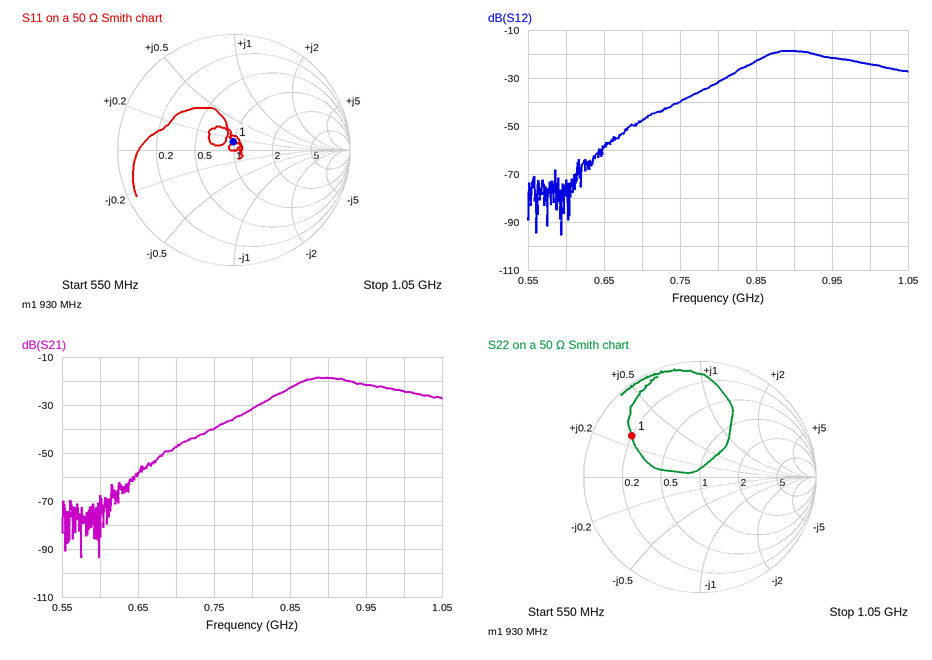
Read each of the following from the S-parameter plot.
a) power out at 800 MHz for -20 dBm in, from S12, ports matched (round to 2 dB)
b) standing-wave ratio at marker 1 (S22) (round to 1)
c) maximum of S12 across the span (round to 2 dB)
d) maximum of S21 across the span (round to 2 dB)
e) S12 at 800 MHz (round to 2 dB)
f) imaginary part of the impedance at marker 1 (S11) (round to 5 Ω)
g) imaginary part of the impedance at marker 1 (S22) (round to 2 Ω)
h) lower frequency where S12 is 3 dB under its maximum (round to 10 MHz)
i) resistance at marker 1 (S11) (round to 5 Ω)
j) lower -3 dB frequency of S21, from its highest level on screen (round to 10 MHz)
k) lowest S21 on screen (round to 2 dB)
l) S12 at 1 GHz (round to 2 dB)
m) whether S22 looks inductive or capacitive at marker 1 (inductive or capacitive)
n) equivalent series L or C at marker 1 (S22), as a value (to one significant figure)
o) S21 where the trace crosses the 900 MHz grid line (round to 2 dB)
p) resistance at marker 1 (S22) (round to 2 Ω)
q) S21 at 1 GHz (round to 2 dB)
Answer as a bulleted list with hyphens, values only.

- -52 dBm
- 5
- -18 dB
- -18 dB
- -32 dB
- +5 Ω
- +14 Ω
- 860 MHz
- 50 Ω
- 860 MHz
- -94 dB
- -24 dB
- inductive
- 2 nH
- -18 dB
- 10 Ω
- -24 dB
